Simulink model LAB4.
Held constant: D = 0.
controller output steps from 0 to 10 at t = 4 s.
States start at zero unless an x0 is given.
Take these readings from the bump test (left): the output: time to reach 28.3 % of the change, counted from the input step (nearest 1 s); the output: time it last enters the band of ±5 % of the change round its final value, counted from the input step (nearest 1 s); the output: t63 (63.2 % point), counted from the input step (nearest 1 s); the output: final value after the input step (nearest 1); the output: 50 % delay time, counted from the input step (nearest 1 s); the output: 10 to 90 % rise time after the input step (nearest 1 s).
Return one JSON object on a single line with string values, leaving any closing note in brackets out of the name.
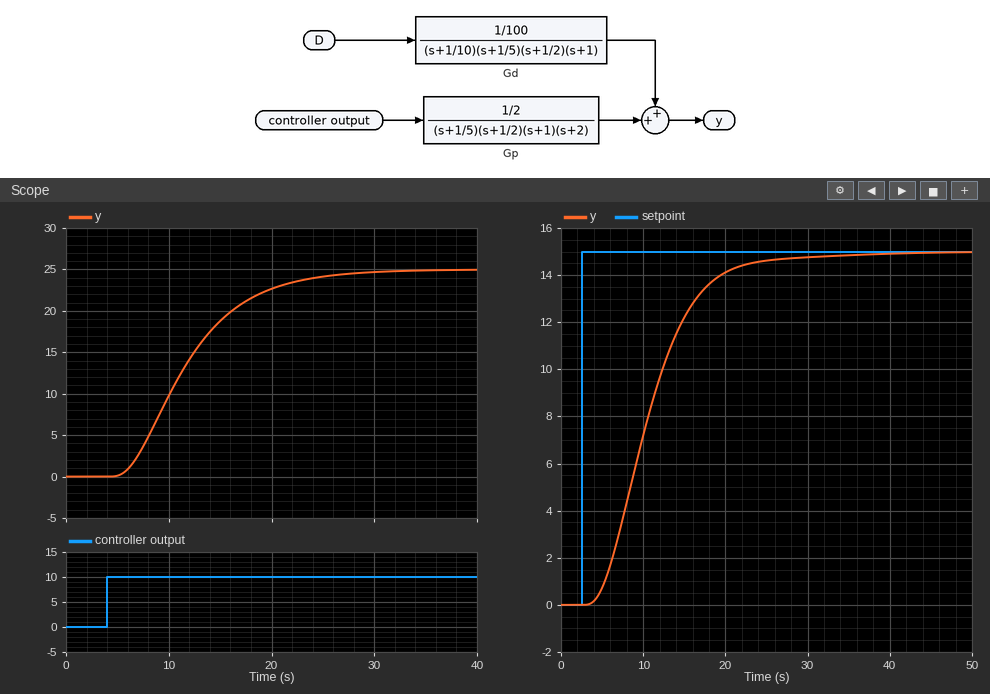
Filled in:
{"the output: time to reach 28.3 % of the change, counted from the input step": "5 s", "the output: time it last enters the band of ±5 % of the change round its final value, counted from the input step": "19 s", "the output: t63 (63.2 % point), counted from the input step": "9 s", "the output: final value after the input step": "25", "the output: 50 % delay time, counted from the input step": "7 s", "the output: 10 to 90 % rise time after the input step": "13 s"}
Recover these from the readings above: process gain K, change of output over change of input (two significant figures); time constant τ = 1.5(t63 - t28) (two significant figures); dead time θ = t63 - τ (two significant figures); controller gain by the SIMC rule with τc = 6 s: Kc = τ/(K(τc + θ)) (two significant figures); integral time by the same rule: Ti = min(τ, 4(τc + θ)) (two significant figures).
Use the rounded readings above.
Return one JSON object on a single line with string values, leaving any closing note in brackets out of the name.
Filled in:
{"process gain K, change of output over change of input": "2.5", "time constant τ = 1.5(t63 - t28)": "6.0 s", "dead time θ = t63 - τ": "3.0 s", "controller gain by the SIMC rule with τc = 6 s: Kc = τ/(K(τc + θ))": "0.27", "integral time by the same rule: Ti = min(τ, 4(τc + θ))": "6.0 s"}
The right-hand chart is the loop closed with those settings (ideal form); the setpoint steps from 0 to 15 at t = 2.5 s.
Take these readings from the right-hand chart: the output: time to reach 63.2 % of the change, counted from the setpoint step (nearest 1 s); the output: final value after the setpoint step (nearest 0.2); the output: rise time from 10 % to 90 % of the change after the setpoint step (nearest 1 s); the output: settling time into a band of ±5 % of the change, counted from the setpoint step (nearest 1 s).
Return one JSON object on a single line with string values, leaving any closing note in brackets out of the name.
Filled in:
{"the output: time to reach 63.2 % of the change, counted from the setpoint step": "9 s", "the output: final value after the setpoint step": "15.0", "the output: rise time from 10 % to 90 % of the change after the setpoint step": "12 s", "the output: settling time into a band of ±5 % of the change, counted from the setpoint step": "18 s"}
